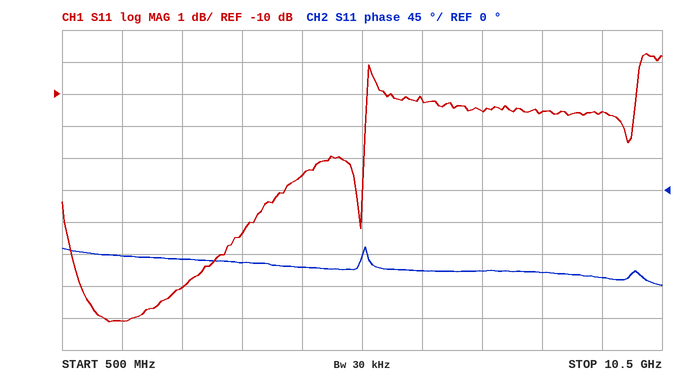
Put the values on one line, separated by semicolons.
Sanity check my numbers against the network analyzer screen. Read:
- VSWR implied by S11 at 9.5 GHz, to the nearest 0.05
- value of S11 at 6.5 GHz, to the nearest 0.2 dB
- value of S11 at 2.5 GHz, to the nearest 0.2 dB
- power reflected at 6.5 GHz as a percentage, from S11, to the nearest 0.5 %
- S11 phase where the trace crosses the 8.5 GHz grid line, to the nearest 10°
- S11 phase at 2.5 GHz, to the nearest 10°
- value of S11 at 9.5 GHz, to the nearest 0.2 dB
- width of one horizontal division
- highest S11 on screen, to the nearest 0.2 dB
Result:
1.85; -10.2 dB; -16.0 dB; 9.5 %; -120°; -100°; -10.6 dB; 1 GHz; -8.8 dB
